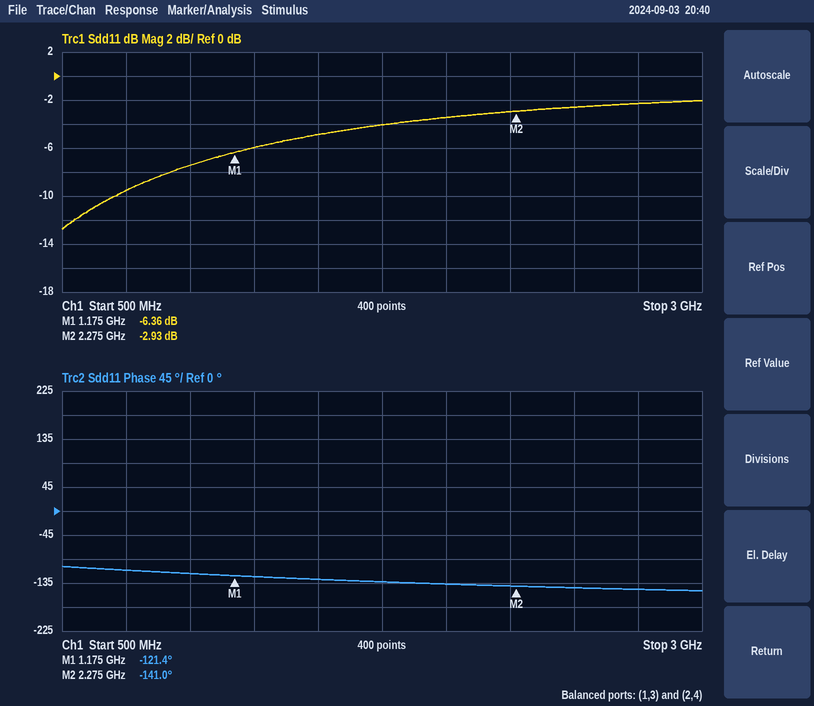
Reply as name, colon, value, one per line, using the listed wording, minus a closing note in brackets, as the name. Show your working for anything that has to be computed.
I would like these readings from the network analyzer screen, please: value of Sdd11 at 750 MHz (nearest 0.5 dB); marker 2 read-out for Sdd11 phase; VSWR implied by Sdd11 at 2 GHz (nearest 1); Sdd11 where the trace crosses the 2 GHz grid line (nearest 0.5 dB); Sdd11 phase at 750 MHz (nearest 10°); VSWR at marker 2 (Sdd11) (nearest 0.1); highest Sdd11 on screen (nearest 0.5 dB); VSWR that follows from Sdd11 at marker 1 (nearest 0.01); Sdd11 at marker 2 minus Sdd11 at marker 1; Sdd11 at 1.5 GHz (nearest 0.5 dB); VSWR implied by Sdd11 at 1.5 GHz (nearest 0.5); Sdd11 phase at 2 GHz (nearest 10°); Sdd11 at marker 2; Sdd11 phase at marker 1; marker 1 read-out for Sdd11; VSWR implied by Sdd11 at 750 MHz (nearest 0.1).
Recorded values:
value of Sdd11 at 750 MHz: -9.5 dB
marker 2 read-out for Sdd11 phase: -141.0°
VSWR implied by Sdd11 at 2 GHz: |Γ| = 10^(-3.5/20) = 0.6683; VSWR = (1 + 0.6683)/(1 − 0.6683) ≈ 5
Sdd11 where the trace crosses the 2 GHz grid line: -3.5 dB
Sdd11 phase at 750 MHz: -110°
VSWR at marker 2 (Sdd11): (1 + 0.7137)/(1 − 0.7137) ≈ 6.0
highest Sdd11 on screen: -2.0 dB
VSWR that follows from Sdd11 at marker 1: (1 + 0.4808)/(1 − 0.4808) ≈ 2.85
Sdd11 at marker 2 minus Sdd11 at marker 1: -2.93 − (-6.36) = 3.43 dB
Sdd11 at 1.5 GHz: -5.0 dB
VSWR implied by Sdd11 at 1.5 GHz: |Γ| = 10^(-5/20) = 0.5623; VSWR = (1 + 0.5623)/(1 − 0.5623) ≈ 3.57, so 3.5 to the nearest 0.5
Sdd11 phase at 2 GHz: -140°
Sdd11 at marker 2: -2.93 dB
Sdd11 phase at marker 1: -121.4°
marker 1 read-out for Sdd11: -6.36 dB
VSWR implied by Sdd11 at 750 MHz: |Γ| = 10^(-9.5/20) = 0.3350; VSWR = (1 + 0.3350)/(1 − 0.3350) ≈ 2.0
